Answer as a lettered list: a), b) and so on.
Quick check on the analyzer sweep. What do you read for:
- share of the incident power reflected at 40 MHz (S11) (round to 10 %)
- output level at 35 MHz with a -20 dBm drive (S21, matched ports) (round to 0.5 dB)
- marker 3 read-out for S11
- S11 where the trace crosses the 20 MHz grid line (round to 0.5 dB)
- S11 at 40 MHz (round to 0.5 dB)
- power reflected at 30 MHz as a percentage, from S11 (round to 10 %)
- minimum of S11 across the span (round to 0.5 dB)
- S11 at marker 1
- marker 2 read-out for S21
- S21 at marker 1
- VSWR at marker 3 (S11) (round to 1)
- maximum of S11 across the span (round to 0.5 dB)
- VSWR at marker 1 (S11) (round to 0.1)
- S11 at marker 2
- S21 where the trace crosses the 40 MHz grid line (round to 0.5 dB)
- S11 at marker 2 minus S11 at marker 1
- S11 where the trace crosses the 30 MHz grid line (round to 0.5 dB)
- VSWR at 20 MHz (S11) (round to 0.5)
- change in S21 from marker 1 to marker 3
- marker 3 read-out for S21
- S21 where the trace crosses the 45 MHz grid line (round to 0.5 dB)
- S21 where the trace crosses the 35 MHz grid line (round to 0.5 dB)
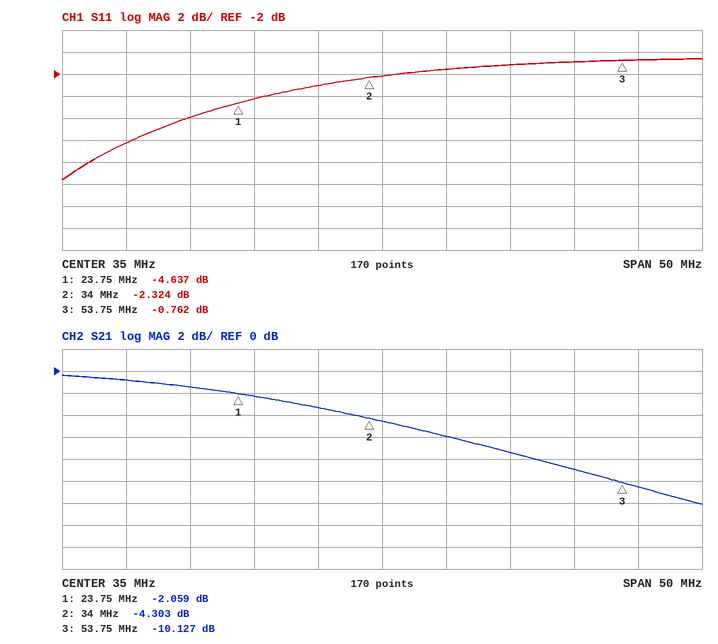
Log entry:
a) 70 %
b) -24.5 dBm
c) -0.762 dB
d) -6.0 dB
e) -1.5 dB
f) 50 %
g) -11.5 dB
h) -4.637 dB
i) -4.303 dB
j) -2.059 dB
k) 23
l) -0.5 dB
m) 3.8
n) -2.324 dB
o) -6.0 dB
p) 2.313 dB
q) -3.0 dB
r) 3.0
s) -8.068 dB
t) -10.127 dB
u) -7.5 dB
v) -4.5 dB
